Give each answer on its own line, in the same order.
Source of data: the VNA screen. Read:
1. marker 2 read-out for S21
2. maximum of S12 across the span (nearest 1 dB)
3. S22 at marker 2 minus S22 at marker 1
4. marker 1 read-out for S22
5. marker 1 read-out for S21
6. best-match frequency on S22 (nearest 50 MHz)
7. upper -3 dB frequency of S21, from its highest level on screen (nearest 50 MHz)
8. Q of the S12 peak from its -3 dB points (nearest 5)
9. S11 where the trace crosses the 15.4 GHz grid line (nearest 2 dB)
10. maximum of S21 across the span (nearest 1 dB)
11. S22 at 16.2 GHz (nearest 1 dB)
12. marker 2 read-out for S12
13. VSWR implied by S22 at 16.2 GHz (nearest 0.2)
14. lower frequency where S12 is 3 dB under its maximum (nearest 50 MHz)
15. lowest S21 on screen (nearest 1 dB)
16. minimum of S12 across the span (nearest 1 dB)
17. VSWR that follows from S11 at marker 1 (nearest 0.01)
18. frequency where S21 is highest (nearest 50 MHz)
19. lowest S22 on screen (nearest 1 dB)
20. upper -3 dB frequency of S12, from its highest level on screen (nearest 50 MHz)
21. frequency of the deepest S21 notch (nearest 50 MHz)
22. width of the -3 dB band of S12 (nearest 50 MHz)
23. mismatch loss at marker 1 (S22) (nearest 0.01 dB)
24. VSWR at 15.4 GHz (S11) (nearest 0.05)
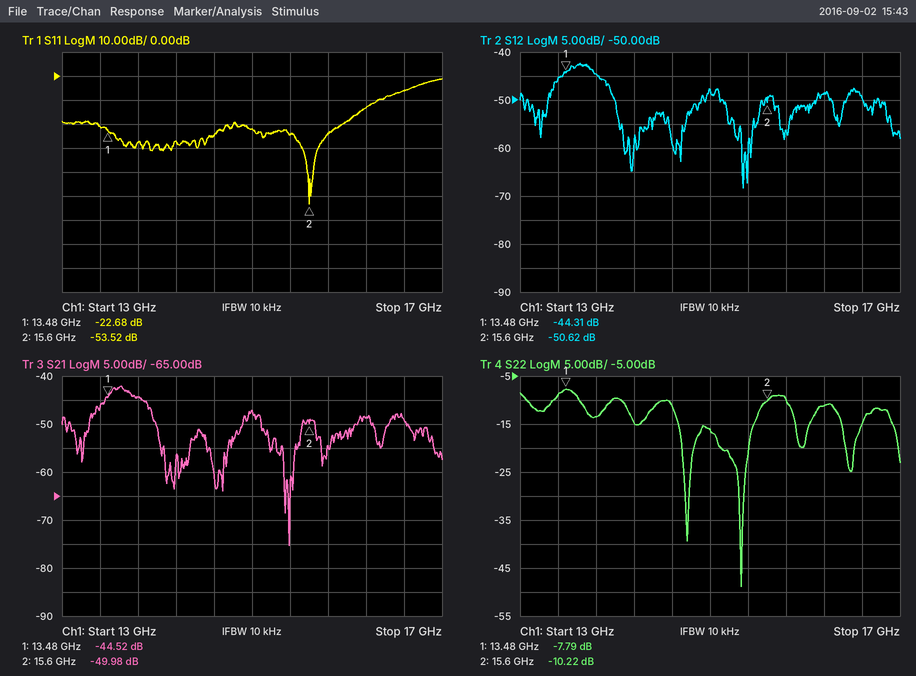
-49.98 dB
-42 dB
-2.43 dB
-7.79 dB
-44.52 dB
15.35 GHz
13.85 GHz
30
-24 dB
-42 dB
-11 dB
-50.62 dB
1.8
13.40 GHz
-75 dB
-68 dB
1.16
13.60 GHz
-49 dB
13.85 GHz
15.40 GHz
450 MHz
0.79 dB
1.15
